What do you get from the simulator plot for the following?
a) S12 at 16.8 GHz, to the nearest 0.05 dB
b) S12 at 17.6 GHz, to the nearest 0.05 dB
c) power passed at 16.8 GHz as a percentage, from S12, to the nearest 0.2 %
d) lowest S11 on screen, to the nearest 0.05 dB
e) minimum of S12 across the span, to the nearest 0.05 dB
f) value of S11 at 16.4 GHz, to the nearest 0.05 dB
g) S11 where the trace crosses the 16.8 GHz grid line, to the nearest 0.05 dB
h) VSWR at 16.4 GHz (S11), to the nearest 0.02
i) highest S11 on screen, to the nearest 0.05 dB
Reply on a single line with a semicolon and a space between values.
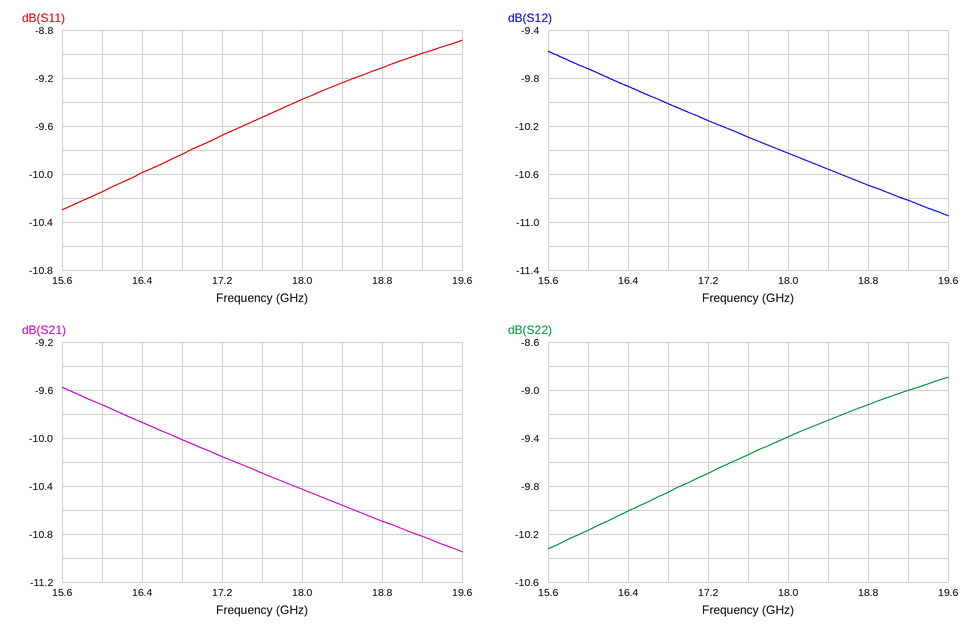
-10.00 dB; -10.30 dB; 10.0 %; -10.30 dB; -10.95 dB; -10.00 dB; -9.85 dB; 1.92; -8.90 dB
